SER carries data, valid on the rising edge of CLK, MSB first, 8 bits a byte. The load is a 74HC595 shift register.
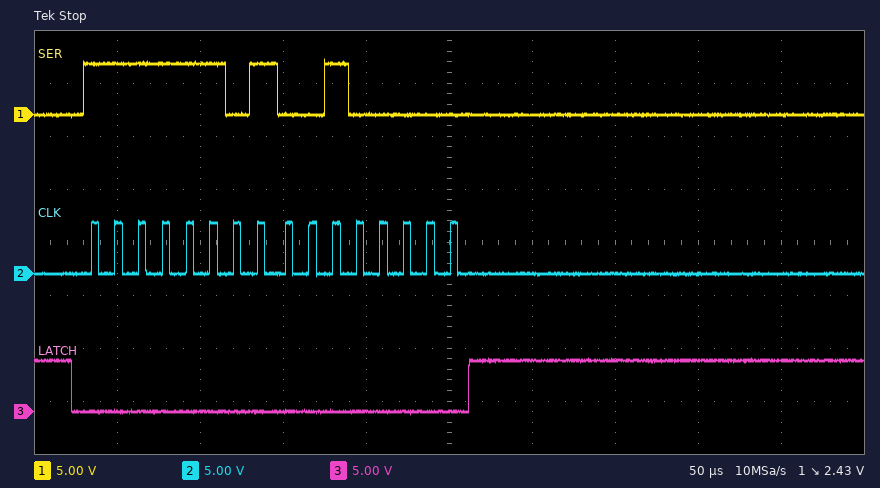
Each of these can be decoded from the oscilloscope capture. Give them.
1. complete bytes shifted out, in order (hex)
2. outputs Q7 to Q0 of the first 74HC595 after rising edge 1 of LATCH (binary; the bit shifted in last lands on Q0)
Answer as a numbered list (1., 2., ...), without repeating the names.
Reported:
1. FD 20
2. 00100000
